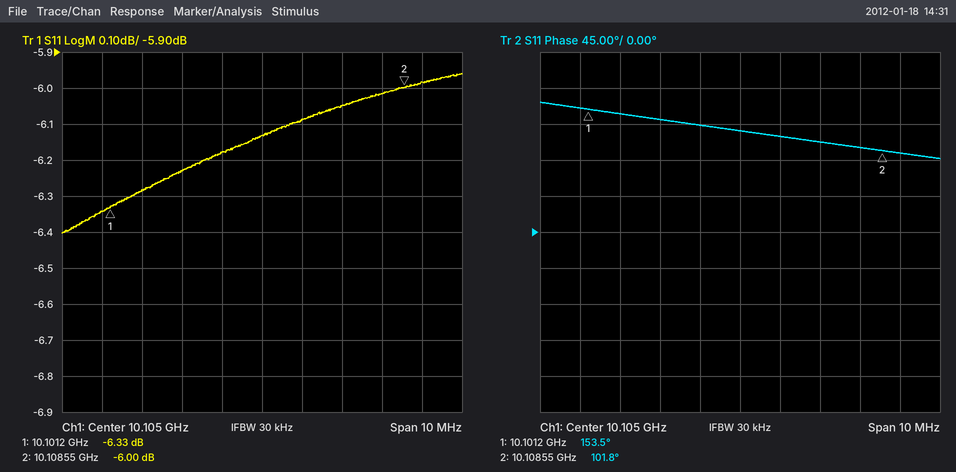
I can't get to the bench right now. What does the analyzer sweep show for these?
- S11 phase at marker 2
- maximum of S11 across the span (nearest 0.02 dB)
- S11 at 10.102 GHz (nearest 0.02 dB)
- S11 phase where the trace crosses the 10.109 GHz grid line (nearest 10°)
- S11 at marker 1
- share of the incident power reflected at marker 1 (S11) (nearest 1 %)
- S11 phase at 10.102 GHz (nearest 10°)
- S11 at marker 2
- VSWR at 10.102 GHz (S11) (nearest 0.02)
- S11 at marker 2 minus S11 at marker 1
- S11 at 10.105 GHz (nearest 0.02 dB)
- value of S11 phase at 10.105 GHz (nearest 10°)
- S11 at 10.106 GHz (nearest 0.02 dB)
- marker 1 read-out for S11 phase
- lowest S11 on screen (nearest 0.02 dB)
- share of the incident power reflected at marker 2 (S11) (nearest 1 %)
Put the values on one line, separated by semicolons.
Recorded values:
101.8°; -5.96 dB; -6.28 dB; 100°; -6.33 dB; 23 %; 150°; -6.00 dB; 2.88; 0.33 dB; -6.14 dB; 130°; -6.08 dB; 153.5°; -6.40 dB; 25 %
